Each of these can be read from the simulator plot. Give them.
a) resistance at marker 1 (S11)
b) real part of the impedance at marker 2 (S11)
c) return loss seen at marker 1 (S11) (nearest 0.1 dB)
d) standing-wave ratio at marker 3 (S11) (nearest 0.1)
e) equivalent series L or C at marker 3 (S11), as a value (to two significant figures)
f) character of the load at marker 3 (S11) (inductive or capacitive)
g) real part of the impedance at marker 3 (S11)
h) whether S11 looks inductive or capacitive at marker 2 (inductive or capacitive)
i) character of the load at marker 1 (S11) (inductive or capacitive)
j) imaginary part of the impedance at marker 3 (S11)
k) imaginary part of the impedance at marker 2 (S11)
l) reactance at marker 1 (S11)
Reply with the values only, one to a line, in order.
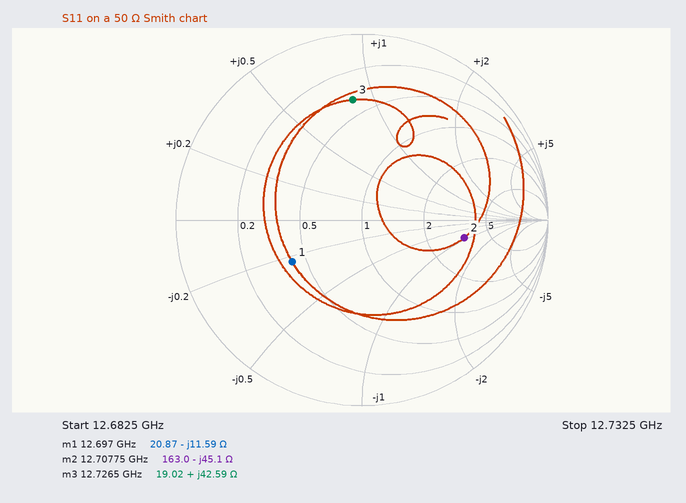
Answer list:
20.87 Ω
163.0 Ω
7.2 dB
4.7
530 pH
inductive
19.02 Ω
capacitive
capacitive
+42.59 Ω
-45.1 Ω
-11.59 Ω
